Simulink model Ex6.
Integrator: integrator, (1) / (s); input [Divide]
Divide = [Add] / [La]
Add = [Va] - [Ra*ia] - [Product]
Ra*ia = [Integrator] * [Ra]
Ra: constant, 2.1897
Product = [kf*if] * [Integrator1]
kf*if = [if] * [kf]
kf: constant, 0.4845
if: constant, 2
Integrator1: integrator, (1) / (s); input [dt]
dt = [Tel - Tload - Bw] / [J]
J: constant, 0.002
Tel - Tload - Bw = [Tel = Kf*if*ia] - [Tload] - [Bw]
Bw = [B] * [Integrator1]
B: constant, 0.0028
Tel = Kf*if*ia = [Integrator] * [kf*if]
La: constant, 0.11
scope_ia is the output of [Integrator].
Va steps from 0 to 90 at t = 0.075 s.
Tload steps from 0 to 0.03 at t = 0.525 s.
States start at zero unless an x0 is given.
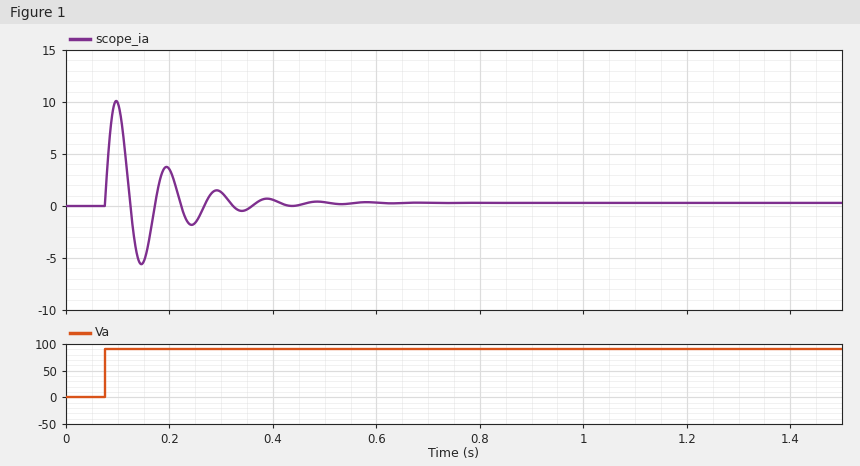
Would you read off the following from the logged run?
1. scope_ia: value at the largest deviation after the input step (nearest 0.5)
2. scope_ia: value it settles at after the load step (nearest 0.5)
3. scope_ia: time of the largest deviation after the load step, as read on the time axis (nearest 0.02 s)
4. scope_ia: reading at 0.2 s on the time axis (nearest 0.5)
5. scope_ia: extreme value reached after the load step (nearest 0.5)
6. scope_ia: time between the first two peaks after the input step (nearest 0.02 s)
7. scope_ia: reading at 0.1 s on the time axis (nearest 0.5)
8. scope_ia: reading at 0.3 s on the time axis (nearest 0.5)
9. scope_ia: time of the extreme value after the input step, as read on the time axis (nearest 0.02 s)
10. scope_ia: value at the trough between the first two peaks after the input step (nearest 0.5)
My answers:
10.0
0.5
0.54 s
3.5
0.0
0.10 s
10.0
1.5
0.10 s
-5.5
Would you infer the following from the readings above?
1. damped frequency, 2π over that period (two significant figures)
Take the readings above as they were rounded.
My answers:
63 rad/s
